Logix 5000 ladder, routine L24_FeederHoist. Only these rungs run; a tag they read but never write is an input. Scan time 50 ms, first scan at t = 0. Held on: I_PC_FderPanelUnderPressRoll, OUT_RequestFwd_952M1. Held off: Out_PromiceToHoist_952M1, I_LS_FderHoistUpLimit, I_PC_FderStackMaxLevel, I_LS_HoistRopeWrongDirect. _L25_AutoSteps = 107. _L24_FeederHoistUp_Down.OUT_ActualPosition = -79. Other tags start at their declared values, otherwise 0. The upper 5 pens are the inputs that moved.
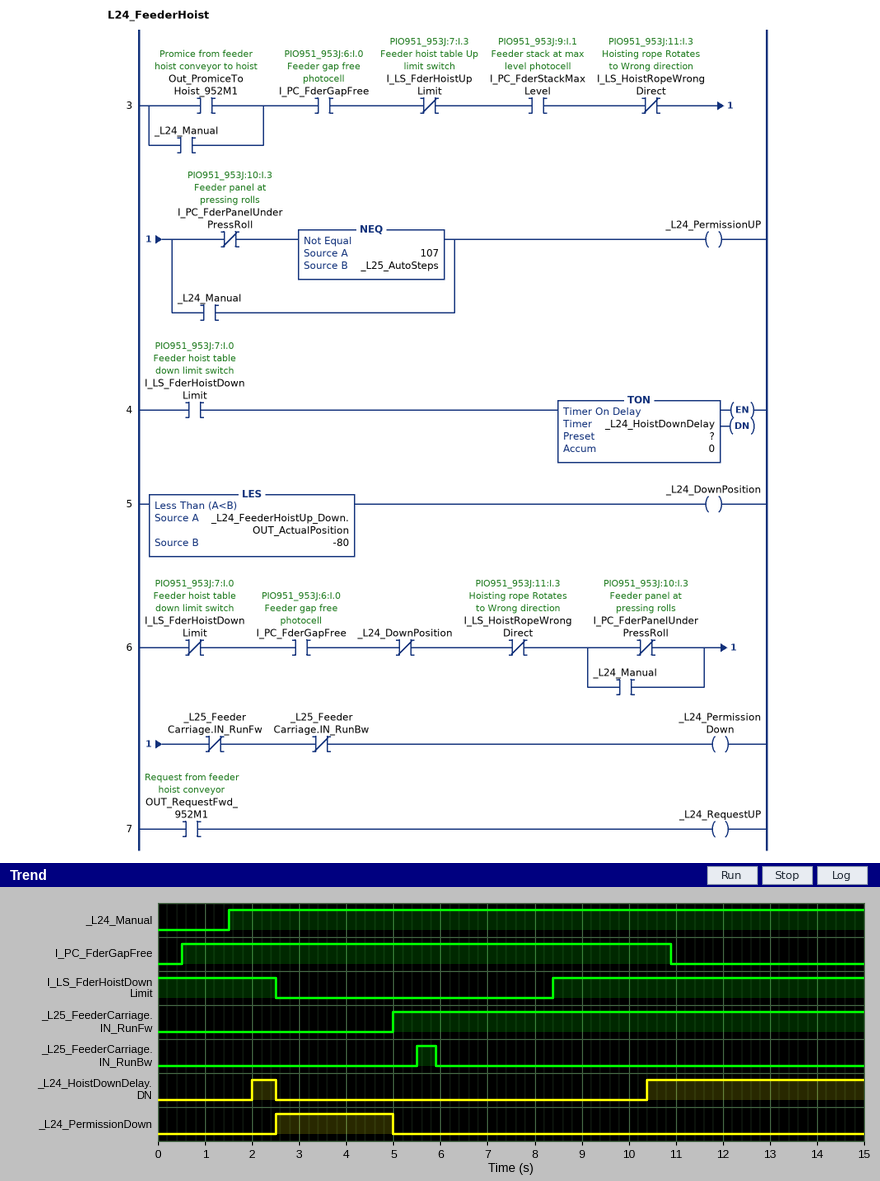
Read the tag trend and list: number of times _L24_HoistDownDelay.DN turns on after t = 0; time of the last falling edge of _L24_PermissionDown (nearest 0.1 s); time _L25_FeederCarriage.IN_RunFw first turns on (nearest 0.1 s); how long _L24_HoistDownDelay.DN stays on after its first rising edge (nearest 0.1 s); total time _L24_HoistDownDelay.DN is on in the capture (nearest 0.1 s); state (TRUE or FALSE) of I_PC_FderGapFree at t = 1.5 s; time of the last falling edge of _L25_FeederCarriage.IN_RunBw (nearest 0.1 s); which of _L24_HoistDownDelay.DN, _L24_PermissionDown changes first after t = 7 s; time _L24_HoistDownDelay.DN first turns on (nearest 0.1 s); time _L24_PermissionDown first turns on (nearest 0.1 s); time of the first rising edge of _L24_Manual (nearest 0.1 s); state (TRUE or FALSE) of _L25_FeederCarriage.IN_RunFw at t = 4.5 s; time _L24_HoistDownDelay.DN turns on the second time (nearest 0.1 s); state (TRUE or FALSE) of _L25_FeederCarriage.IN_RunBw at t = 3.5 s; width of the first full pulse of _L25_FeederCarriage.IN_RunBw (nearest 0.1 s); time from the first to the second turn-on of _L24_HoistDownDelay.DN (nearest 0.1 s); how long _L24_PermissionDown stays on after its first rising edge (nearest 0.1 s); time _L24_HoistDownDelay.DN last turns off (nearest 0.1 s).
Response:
2
5.0 s
5.0 s
0.5 s
5.1 s
TRUE
5.9 s
_L24_HoistDownDelay.DN
2.0 s
2.5 s
1.5 s
FALSE
10.4 s
FALSE
0.4 s
8.4 s
2.5 s
2.5 s
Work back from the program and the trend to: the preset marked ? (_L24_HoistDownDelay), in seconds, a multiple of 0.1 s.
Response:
2.0 s
